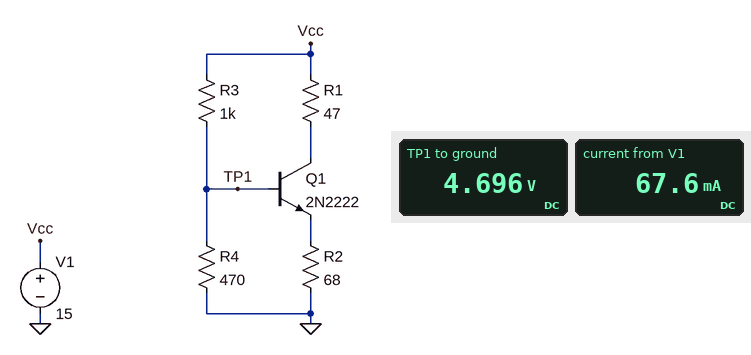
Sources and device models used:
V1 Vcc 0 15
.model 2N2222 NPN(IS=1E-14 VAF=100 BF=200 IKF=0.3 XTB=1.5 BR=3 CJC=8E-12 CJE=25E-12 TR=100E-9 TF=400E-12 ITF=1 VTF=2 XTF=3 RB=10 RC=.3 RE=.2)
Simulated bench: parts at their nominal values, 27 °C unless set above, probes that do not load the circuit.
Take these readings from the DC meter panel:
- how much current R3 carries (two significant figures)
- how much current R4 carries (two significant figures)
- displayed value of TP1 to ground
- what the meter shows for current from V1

10 mA
10 mA
4.696 V
67.6 mA
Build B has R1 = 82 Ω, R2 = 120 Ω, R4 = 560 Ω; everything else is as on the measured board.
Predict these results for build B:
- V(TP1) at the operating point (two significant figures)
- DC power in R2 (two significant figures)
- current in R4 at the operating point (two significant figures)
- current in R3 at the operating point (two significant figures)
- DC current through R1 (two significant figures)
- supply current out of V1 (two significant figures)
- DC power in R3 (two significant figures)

5.3 V
170 mW
9.5 mA
9.7 mA
38 mA
47 mA
94 mW
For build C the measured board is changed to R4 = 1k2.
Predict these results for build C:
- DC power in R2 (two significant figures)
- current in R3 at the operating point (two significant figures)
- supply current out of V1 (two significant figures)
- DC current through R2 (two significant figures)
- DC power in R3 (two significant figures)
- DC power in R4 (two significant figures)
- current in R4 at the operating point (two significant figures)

720 mW
7.2 mA
110 mA
100 mA
52 mW
51 mW
6.5 mA
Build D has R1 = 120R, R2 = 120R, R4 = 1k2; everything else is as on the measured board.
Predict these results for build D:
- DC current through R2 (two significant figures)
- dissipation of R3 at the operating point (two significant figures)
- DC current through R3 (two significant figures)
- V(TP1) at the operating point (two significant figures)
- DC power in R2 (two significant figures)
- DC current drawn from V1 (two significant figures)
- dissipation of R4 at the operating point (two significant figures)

60 mA
49 mW
7.0 mA
8.0 V
430 mW
67 mA
53 mW
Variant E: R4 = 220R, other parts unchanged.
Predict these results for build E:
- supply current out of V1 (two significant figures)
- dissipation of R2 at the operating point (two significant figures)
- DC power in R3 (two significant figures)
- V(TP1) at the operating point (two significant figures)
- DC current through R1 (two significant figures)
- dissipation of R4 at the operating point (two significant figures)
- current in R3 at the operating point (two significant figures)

41 mA
55 mW
150 mW
2.7 V
28 mA
33 mW
12 mA
